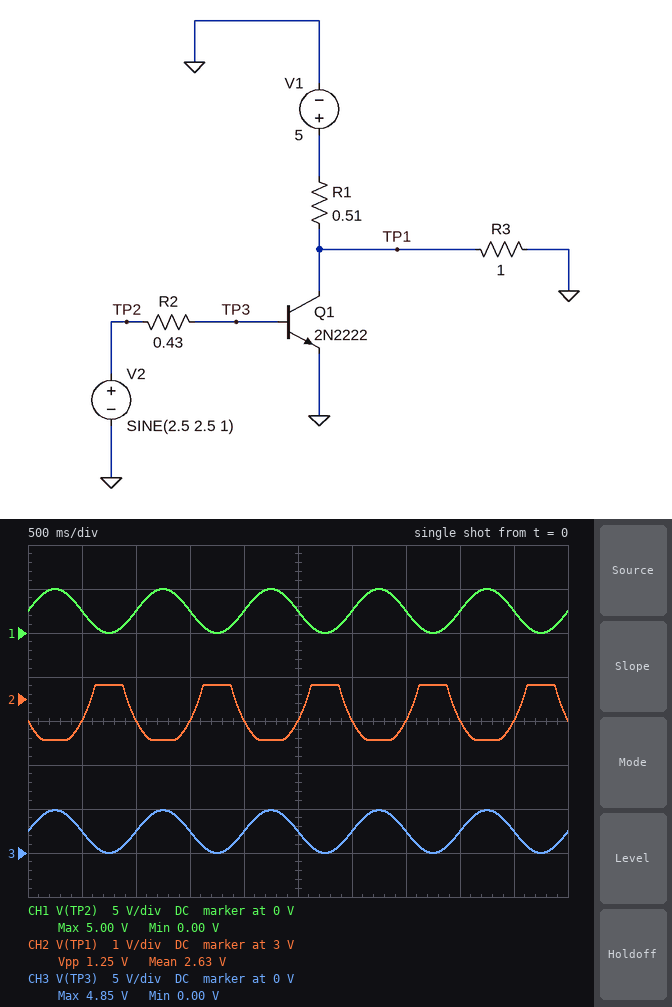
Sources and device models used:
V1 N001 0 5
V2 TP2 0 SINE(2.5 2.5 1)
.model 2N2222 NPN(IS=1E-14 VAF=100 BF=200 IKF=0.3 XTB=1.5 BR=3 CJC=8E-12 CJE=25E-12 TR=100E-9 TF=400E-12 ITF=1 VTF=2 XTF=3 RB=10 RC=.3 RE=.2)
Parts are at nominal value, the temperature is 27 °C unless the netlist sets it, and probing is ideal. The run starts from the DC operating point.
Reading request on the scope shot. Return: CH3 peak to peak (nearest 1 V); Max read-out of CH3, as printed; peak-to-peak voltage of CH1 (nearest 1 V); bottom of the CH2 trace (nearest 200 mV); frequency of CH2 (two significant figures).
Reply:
5 V
4.85 V
5 V
2.0 V
1.0 Hz
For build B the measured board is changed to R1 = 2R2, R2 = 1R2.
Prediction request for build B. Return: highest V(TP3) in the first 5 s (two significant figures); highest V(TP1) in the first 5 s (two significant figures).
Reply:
4.6 V
1.6 V
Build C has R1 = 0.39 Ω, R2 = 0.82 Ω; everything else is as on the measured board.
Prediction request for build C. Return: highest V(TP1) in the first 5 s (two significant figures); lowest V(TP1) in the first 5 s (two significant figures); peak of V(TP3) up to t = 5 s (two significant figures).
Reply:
3.6 V
2.5 V
4.8 V
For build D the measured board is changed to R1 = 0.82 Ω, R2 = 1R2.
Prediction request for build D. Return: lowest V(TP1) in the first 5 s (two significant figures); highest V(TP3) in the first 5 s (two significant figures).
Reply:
1.5 V
4.6 V
